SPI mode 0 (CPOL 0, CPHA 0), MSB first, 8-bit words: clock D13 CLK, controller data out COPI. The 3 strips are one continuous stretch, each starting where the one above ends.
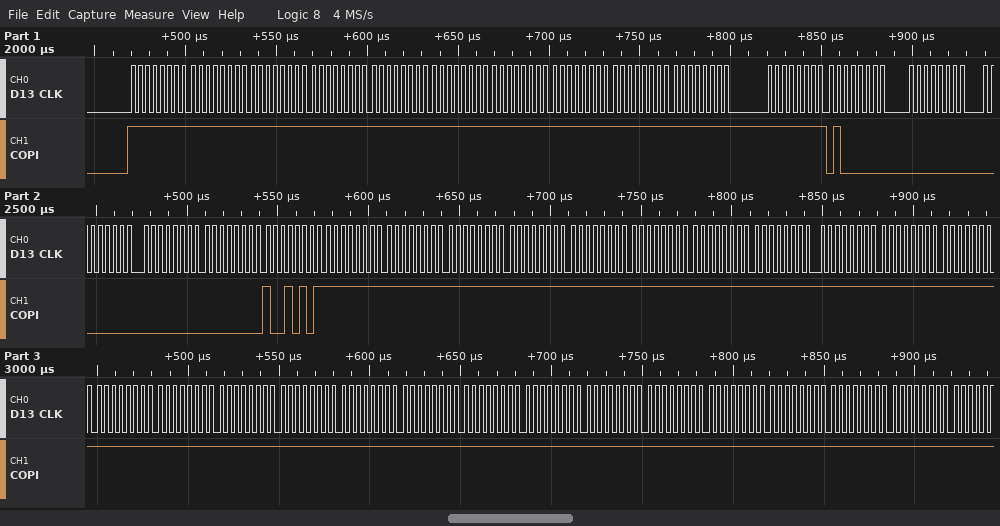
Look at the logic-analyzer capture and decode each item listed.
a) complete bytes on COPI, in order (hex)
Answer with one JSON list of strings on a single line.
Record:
["FF FF FF FF FF FF FF FF FF FF FF 40 00 00 00 00 95 FF FF FF FF FF FF FF FF FF FF FF FF FF FF FF FF FF FF FF FF FF FF FF FF FF"]
